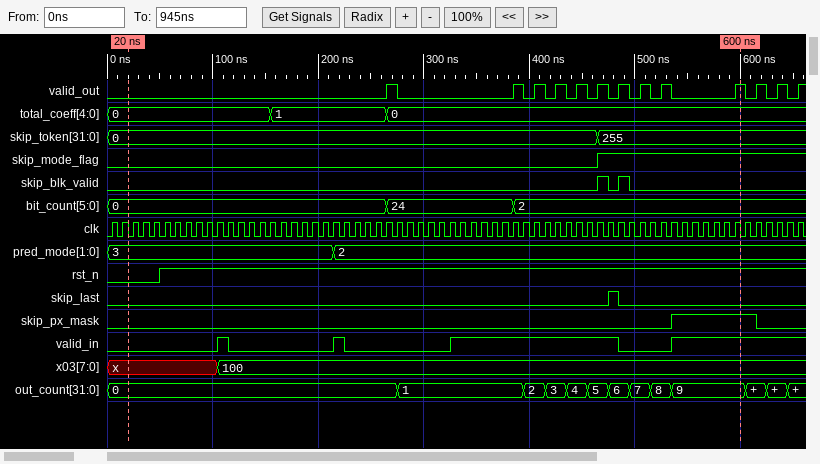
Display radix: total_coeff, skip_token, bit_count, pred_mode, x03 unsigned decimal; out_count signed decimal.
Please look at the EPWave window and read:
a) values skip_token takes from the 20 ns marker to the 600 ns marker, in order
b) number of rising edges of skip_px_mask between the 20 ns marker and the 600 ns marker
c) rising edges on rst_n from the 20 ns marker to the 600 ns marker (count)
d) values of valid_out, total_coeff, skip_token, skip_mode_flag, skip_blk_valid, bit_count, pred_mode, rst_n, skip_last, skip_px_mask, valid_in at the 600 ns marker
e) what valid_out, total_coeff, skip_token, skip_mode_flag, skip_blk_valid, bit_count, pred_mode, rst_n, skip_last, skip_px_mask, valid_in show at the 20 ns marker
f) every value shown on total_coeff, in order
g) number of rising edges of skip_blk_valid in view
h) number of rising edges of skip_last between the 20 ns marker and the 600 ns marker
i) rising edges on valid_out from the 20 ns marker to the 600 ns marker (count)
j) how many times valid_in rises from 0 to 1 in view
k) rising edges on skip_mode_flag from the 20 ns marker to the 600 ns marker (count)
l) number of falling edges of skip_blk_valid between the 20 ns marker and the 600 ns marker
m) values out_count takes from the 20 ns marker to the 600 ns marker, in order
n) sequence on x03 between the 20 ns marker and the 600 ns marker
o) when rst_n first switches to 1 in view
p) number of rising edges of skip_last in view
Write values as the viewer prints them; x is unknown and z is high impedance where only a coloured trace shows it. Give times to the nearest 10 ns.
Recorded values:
0, 255
1
1
valid_out=1, total_coeff=0, skip_token=255, skip_mode_flag=1, skip_blk_valid=0, bit_count=2, pred_mode=2, rst_n=1, skip_last=0, skip_px_mask=1, valid_in=1
valid_out=0, total_coeff=0, skip_token=0, skip_mode_flag=0, skip_blk_valid=0, bit_count=0, pred_mode=3, rst_n=0, skip_last=0, skip_px_mask=0, valid_in=0
0, 1, 0
2
1
10
4
1
2
0, 1, 2, 3, 4, 5, 6, 7, 8, 9
x, 100
50 ns
1
